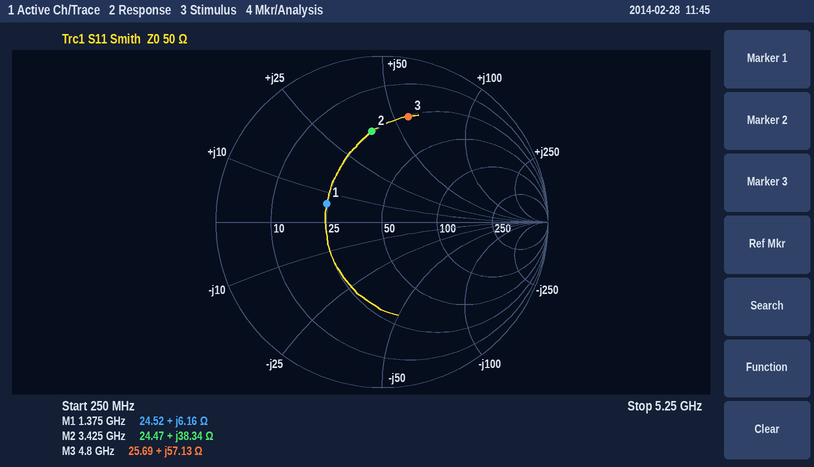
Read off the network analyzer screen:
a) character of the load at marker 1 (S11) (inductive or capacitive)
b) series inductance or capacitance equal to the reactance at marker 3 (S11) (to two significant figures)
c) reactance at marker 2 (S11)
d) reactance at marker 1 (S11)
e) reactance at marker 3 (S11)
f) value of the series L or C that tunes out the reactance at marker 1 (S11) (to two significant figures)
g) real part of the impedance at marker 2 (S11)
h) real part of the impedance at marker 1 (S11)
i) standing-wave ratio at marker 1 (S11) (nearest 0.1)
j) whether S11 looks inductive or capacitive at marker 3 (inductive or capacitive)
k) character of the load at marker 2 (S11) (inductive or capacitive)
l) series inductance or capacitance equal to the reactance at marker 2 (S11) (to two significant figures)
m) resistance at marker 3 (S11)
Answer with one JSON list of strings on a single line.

["inductive", "1.9 nH", "+38.34 Ω", "+6.16 Ω", "+57.13 Ω", "19 pF", "24.47 Ω", "24.52 Ω", "2.1", "inductive", "inductive", "1.8 nH", "25.69 Ω"]
